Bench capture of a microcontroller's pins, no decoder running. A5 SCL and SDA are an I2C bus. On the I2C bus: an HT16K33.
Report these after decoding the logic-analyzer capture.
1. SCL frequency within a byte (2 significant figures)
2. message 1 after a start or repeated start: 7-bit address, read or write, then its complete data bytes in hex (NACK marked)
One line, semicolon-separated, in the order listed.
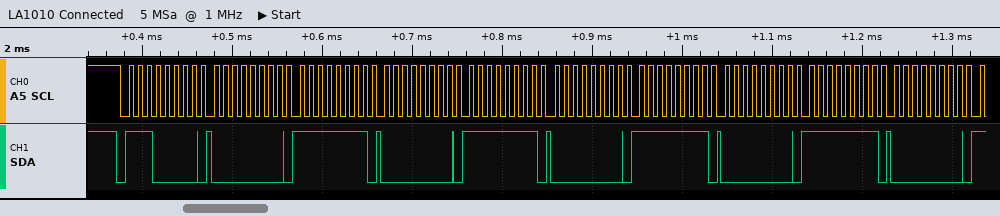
100 kHz; 0x70 write: 00 FF 00 FF 00 FF 00 FF 00
